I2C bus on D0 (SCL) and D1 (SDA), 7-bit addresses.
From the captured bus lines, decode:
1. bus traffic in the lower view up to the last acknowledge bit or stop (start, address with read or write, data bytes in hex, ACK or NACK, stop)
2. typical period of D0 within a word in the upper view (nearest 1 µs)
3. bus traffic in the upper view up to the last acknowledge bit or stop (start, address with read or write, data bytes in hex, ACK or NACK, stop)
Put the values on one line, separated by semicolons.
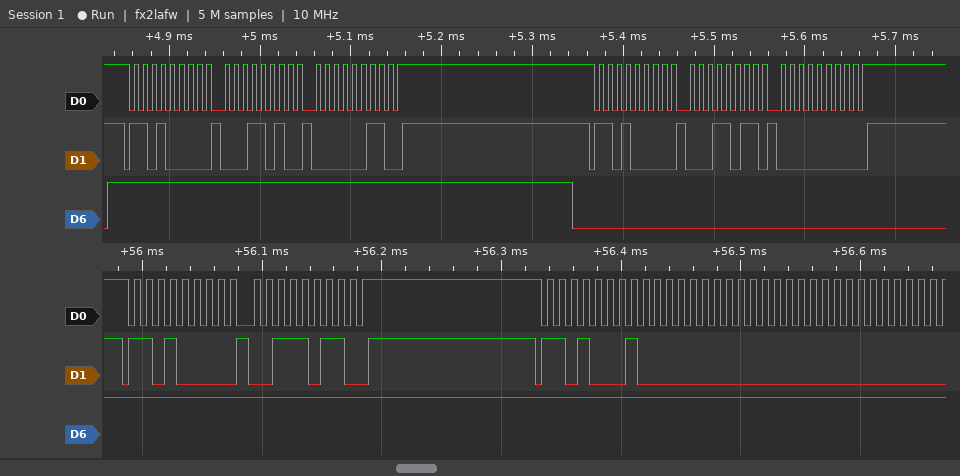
start, address 68 write ACK, 3B ACK, stop, start, address 68 read ACK, 00 ACK, 00 ACK; 10 µs; start, address 68 write ACK, 1A ACK, 03 ACK, stop, start, address 68 write ACK, 1B ACK, 00 ACK, stop
